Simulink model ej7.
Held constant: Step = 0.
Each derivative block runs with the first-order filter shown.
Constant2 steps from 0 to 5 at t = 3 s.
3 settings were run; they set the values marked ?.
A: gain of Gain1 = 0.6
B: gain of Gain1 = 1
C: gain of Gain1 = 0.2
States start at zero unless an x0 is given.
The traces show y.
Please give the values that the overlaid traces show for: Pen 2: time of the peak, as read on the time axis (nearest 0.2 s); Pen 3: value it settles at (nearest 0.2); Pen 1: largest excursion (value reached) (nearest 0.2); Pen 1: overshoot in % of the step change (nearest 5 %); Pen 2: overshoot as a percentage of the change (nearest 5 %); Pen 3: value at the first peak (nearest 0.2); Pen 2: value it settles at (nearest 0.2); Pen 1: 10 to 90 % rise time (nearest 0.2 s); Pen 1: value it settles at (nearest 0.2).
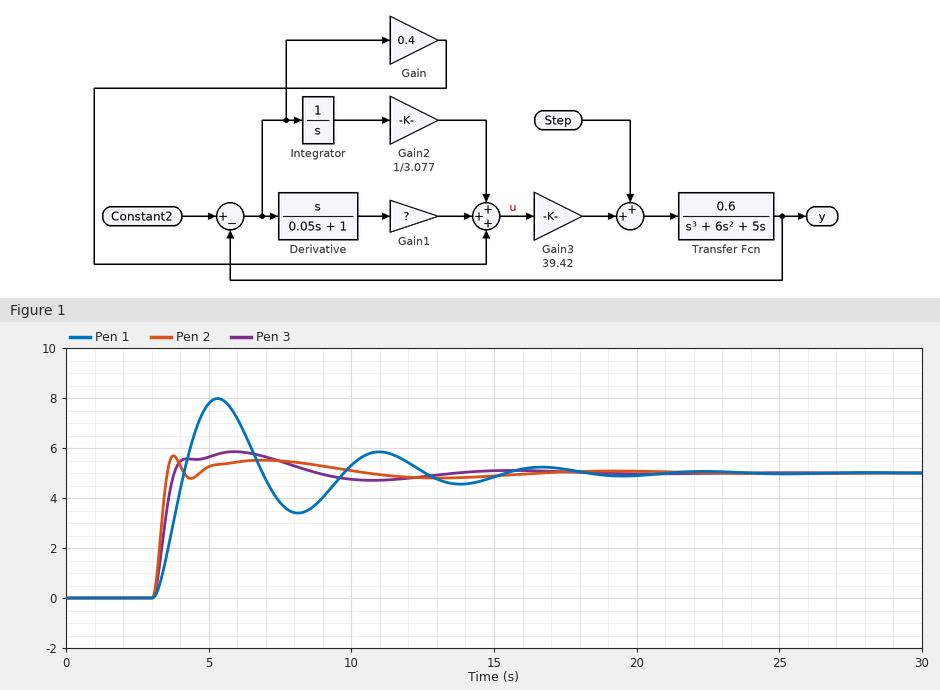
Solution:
3.8 s
5.0
8.0
60 %
15 %
5.8
5.0
0.8 s
5.0
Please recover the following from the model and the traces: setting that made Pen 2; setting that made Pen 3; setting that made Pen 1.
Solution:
B
A
C
